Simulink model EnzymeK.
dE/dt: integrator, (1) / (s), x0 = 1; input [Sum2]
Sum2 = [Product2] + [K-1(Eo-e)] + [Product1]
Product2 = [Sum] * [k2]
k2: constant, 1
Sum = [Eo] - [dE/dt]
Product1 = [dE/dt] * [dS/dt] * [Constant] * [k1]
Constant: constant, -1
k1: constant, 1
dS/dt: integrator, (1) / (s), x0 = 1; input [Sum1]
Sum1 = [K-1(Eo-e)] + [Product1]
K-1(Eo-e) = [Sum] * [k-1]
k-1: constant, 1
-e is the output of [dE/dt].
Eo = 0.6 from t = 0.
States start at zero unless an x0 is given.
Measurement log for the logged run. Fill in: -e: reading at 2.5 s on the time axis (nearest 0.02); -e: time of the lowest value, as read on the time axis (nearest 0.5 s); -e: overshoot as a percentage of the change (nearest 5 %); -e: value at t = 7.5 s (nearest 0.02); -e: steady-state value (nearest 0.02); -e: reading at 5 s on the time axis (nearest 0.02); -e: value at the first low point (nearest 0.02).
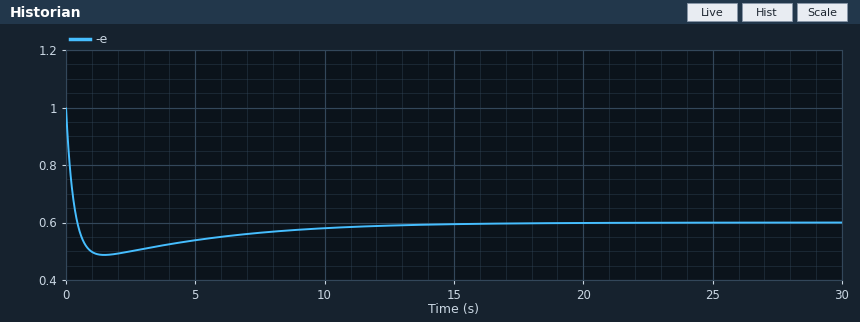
0.50
1.5 s
30 %
0.56
0.60
0.54
0.48
